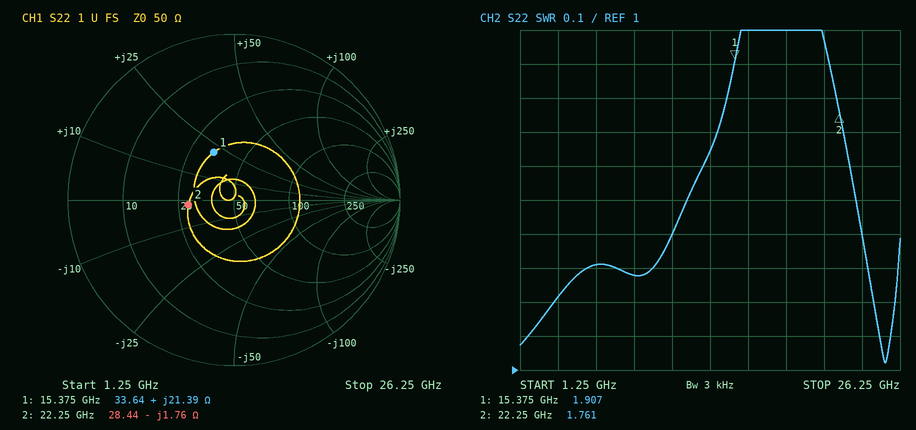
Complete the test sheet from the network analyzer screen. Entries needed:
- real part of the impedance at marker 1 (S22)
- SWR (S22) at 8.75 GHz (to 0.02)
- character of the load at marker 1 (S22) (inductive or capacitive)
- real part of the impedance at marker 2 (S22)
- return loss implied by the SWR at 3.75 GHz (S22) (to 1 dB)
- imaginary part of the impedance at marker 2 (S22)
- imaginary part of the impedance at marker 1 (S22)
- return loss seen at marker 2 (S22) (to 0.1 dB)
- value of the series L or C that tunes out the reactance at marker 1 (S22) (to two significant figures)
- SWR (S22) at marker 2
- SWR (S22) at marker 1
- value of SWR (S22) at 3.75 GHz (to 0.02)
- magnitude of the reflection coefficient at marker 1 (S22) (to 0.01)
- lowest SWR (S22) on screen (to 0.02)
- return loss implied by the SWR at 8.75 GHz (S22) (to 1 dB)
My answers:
33.64 Ω
1.28
inductive
28.44 Ω
20 dB
-1.76 Ω
+21.39 Ω
11.2 dB
480 fF
1.761
1.907
1.22
0.31
1.02
18 dB
